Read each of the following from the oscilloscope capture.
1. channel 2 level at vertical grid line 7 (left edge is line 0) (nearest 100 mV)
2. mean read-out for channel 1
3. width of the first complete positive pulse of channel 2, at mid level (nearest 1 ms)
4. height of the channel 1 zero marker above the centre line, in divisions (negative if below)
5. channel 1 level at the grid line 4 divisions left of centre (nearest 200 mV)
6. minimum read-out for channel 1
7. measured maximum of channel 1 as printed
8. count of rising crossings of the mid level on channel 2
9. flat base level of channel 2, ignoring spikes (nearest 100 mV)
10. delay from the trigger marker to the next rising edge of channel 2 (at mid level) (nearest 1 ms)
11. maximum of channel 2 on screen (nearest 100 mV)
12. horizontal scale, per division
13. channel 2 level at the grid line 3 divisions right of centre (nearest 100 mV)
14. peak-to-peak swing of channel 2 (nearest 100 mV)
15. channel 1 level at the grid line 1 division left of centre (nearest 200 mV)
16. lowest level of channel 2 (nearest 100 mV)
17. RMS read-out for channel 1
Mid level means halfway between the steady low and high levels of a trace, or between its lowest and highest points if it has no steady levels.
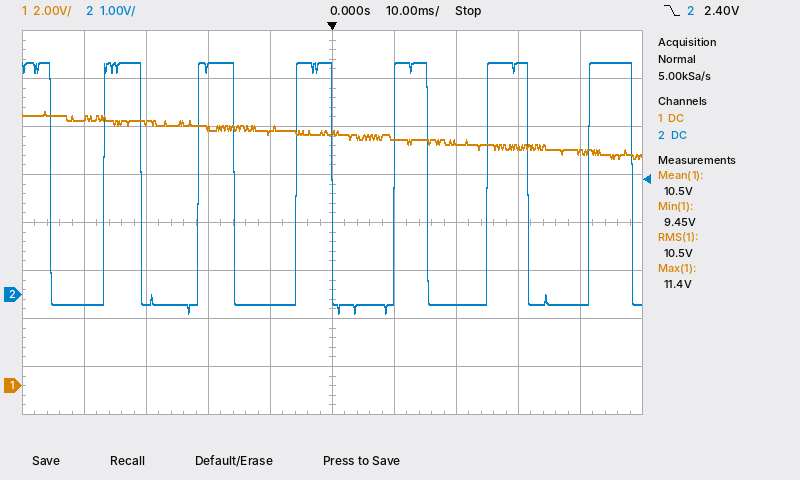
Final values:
-200 mV
10.5 V
6 ms
-3.4 div
11.2 V
9.45 V
11.4 V
6
-200 mV
10 ms
4.8 V
10 ms
4.8 V
5.2 V
10.6 V
-400 mV
10.5 V
